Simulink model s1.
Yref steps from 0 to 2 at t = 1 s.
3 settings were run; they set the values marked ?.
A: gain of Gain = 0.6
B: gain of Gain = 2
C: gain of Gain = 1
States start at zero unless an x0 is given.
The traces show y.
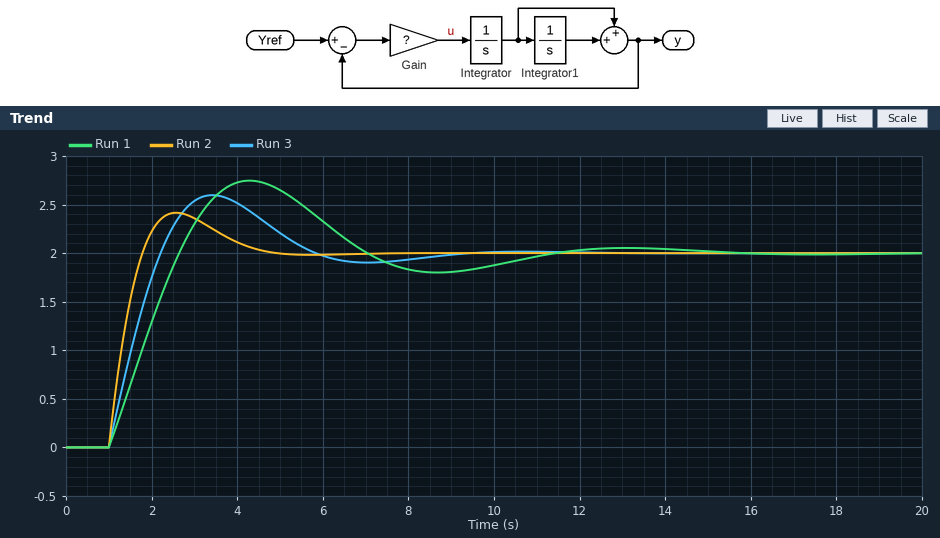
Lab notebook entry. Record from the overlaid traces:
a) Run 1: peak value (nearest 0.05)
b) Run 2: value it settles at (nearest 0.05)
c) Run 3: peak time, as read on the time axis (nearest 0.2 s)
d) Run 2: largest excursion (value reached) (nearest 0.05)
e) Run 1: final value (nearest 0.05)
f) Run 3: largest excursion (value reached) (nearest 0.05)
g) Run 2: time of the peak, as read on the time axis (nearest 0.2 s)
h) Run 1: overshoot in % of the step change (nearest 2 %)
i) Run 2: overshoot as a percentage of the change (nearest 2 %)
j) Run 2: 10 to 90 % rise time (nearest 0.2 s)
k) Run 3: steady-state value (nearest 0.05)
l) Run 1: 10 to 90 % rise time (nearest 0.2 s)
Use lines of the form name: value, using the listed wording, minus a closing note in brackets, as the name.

Run 1: peak value: 2.75
Run 2: value it settles at: 2.00
Run 3: peak time, as read on the time axis: 3.4 s
Run 2: largest excursion (value reached): 2.40
Run 1: final value: 2.00
Run 3: largest excursion (value reached): 2.60
Run 2: time of the peak, as read on the time axis: 2.6 s
Run 1: overshoot in % of the step change: 38 %
Run 2: overshoot as a percentage of the change: 20 %
Run 2: 10 to 90 % rise time: 0.6 s
Run 3: steady-state value: 2.00
Run 1: 10 to 90 % rise time: 1.2 s
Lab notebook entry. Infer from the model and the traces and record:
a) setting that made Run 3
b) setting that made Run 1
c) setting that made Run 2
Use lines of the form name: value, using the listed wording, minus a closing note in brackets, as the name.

setting that made Run 3: C
setting that made Run 1: A
setting that made Run 2: B
